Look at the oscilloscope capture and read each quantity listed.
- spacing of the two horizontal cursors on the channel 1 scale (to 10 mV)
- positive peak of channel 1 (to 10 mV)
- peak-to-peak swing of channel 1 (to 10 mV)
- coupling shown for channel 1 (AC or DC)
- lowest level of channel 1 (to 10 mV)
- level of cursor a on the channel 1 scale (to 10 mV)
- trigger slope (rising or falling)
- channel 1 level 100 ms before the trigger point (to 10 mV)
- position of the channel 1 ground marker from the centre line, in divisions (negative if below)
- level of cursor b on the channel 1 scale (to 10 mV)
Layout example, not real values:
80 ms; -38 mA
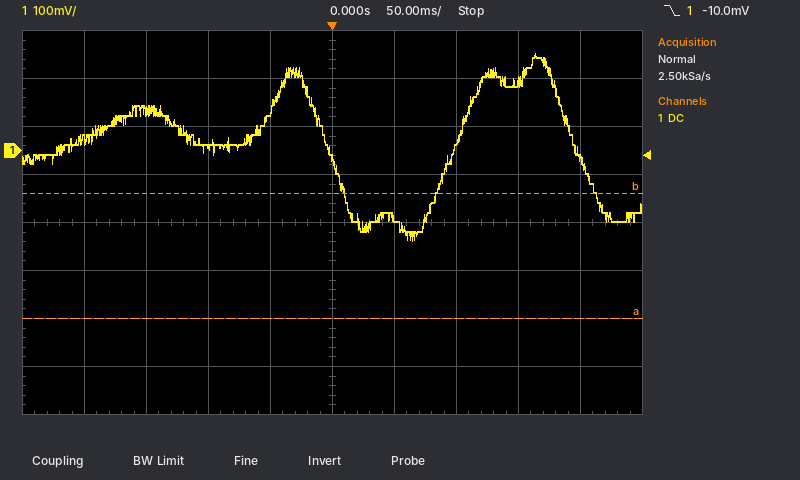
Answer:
260 mV; 200 mV; 390 mV; DC; -190 mV; -350 mV; falling; 10 mV; +1.5 div; -90 mV
